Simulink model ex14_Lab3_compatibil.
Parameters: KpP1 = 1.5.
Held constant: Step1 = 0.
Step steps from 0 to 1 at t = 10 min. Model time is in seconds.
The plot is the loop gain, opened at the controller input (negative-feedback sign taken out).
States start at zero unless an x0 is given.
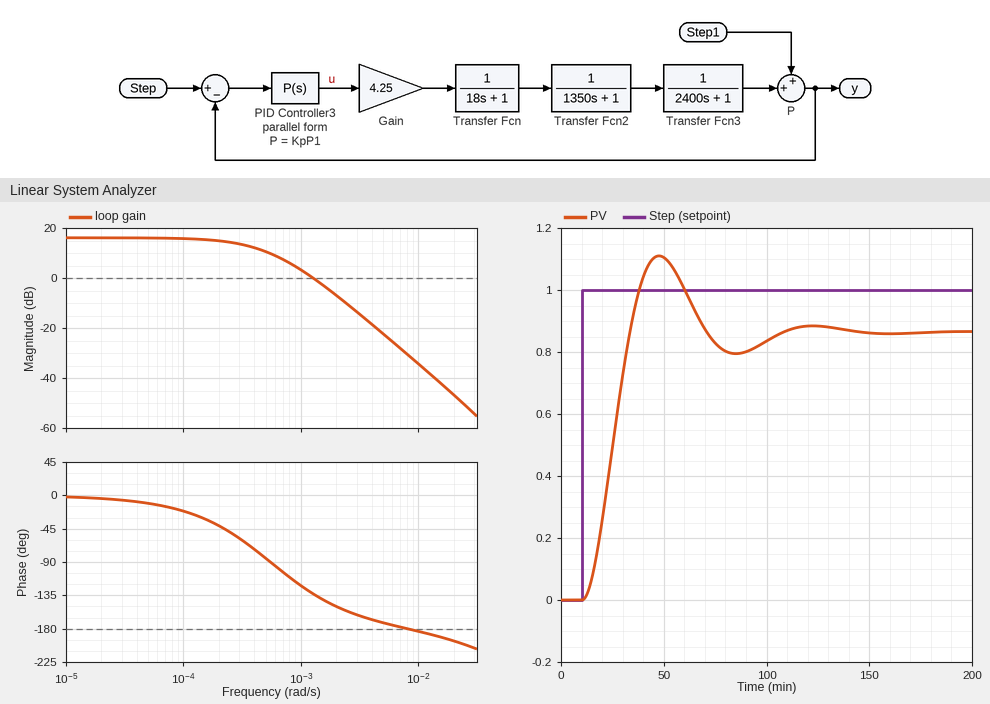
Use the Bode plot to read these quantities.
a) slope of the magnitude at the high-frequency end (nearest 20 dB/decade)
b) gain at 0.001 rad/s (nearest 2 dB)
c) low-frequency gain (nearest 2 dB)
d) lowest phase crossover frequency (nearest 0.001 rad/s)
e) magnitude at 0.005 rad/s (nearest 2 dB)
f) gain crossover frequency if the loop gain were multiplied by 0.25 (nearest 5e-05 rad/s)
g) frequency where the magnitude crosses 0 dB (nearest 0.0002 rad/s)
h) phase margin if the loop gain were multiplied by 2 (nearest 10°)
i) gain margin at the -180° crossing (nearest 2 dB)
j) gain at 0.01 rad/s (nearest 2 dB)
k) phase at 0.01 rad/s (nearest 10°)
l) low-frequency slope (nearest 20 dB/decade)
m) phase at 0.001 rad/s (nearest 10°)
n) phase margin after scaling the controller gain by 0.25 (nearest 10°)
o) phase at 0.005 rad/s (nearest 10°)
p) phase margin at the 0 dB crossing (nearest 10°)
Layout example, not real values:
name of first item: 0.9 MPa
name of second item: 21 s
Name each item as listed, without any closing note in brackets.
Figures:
slope of the magnitude at the high-frequency end: -40 dB/decade
gain at 0.001 rad/s: 4 dB
low-frequency gain: 16 dB
lowest phase crossover frequency: 0.008 rad/s
magnitude at 0.005 rad/s: -22 dB
gain crossover frequency if the loop gain were multiplied by 0.25: 0.00040 rad/s
frequency where the magnitude crosses 0 dB: 0.0012 rad/s
phase margin if the loop gain were multiplied by 2: 30°
gain margin at the -180° crossing: 30 dB
gain at 0.01 rad/s: -34 dB
phase at 0.01 rad/s: -180°
low-frequency slope: 0 dB/decade
phase at 0.001 rad/s: -120°
phase margin after scaling the controller gain by 0.25: 110°
phase at 0.005 rad/s: -170°
phase margin at the 0 dB crossing: 50°
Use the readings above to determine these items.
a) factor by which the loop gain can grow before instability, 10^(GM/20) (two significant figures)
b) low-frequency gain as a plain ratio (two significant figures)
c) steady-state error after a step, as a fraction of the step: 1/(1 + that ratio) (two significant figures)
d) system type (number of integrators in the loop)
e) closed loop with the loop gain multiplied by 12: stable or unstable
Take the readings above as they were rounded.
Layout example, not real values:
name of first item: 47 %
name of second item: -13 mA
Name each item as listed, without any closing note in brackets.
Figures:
factor by which the loop gain can grow before instability, 10^(GM/20): 32
low-frequency gain as a plain ratio: 6.3
steady-state error after a step, as a fraction of the step: 1/(1 + that ratio): 0.14
system type: 0
closed loop with the loop gain multiplied by 12: stable or unstable: stable
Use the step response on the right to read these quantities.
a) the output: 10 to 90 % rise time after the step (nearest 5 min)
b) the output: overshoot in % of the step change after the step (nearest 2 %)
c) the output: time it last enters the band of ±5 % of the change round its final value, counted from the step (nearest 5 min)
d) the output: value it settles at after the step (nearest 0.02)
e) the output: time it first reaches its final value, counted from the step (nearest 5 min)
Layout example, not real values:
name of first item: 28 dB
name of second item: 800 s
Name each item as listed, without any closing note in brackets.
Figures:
the output: 10 to 90 % rise time after the step: 15 min
the output: overshoot in % of the step change after the step: 28 %
the output: time it last enters the band of ±5 % of the change round its final value, counted from the step: 85 min
the output: value it settles at after the step: 0.86
the output: time it first reaches its final value, counted from the step: 25 min
